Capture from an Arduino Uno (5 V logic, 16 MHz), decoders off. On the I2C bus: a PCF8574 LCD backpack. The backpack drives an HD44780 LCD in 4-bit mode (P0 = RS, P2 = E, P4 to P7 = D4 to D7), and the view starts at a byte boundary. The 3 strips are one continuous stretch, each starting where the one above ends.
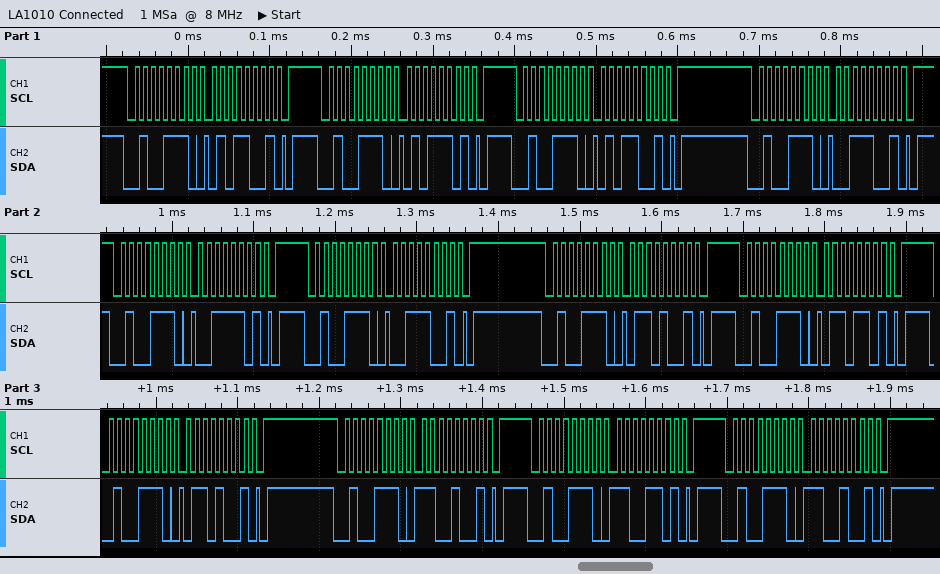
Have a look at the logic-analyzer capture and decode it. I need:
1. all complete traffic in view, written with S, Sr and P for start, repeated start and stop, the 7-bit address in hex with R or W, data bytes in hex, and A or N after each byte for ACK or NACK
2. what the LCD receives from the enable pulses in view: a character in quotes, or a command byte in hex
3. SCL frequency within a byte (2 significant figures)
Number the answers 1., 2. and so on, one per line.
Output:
1. S 27W A 59 A P S 27W A 5D A P S 27W A 59 A P S 27W A 39 A P S 27W A 3D A P S 27W A 39 A P S 27W A 69 A P S 27W A 6D A P S 27W A 69 A P S 27W A C9 A P S 27W A CD A P S 27W A C9 A P
2. 'S' 'l'
3. 100 kHz
